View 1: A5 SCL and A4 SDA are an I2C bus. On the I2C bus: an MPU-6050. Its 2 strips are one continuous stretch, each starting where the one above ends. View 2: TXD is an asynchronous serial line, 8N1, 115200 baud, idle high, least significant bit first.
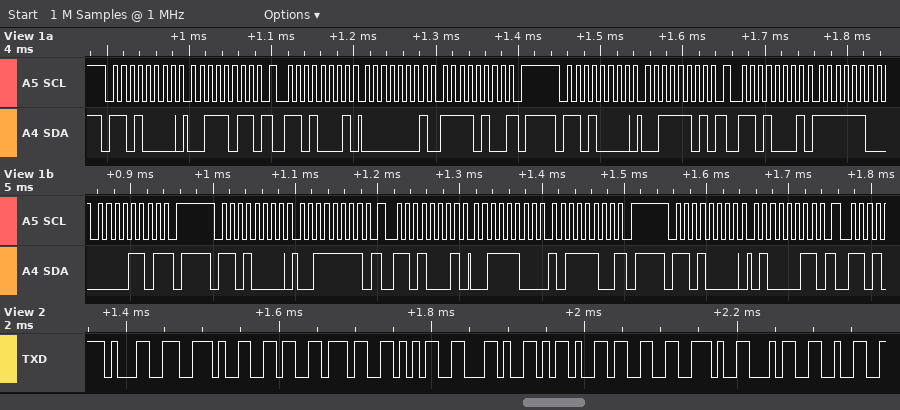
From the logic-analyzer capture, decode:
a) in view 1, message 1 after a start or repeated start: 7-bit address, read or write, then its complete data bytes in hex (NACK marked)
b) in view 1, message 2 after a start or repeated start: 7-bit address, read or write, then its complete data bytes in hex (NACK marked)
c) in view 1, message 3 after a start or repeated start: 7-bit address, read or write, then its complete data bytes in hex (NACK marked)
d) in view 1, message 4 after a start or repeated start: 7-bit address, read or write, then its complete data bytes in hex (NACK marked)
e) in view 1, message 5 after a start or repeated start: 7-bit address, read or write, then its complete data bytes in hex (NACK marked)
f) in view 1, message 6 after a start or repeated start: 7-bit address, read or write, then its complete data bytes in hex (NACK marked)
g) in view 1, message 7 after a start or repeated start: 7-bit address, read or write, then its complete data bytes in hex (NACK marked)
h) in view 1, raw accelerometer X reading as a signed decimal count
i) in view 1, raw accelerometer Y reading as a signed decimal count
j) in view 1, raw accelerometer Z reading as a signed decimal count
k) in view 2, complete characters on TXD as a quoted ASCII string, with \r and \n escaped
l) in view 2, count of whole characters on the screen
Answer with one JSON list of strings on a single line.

["0x68 write: 3B", "0x68 read: 01 F4 NACK", "0x68 write: 3D", "0x68 read: FC 0D NACK", "0x68 write: 3F", "0x68 read: 3C BC NACK", "0x68 write: 43", "500", "-1011", "15548", "\"1.675,-3.42\"", "11"]
